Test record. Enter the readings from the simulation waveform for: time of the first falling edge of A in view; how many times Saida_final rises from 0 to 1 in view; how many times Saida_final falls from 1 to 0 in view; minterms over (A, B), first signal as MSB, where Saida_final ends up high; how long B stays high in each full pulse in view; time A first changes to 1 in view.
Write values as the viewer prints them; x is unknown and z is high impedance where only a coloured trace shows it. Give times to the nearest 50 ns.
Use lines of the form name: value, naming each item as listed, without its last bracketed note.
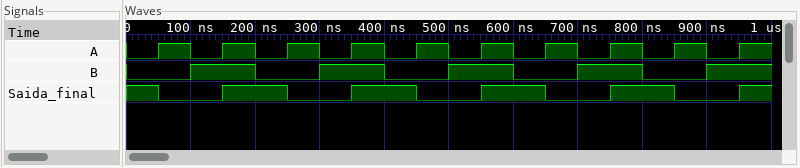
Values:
time of the first falling edge of A in view: 100 ns
how many times Saida_final rises from 0 to 1 in view: 5
how many times Saida_final falls from 1 to 0 in view: 5
minterms over (A, B), first signal as MSB, where Saida_final ends up high: 0, 3
how long B stays high in each full pulse in view: 100 ns, 100 ns, 100 ns, 100 ns
time A first changes to 1 in view: 50 ns
